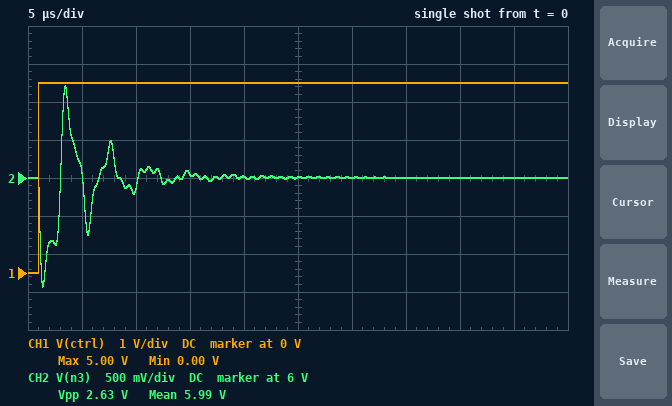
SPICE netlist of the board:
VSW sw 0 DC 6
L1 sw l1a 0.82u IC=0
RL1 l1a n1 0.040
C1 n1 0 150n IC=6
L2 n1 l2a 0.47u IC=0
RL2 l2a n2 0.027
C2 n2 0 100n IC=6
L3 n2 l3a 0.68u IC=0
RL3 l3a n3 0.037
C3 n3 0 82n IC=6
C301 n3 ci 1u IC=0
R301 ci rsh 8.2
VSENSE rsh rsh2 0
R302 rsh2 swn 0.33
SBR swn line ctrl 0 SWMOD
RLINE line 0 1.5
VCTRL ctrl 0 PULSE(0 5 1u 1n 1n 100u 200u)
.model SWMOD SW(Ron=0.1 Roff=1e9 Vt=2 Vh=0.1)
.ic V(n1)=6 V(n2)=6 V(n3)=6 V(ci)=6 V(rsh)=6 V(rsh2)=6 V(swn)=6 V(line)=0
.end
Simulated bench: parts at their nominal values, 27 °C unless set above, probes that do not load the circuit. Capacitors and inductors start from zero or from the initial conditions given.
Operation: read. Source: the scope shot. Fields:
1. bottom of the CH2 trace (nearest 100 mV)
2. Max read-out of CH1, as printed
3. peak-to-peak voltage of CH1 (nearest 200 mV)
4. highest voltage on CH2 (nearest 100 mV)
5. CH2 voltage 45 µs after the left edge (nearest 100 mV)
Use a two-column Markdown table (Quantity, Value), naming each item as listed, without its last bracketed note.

| Quantity | Value |
|---|---|
| bottom of the CH2 trace | 4.6 V |
| Max read-out of CH1, as printed | 5.00 V |
| peak-to-peak voltage of CH1 | 5.0 V |
| highest voltage on CH2 | 7.2 V |
| CH2 voltage 45 µs after the left edge | 6.0 V |
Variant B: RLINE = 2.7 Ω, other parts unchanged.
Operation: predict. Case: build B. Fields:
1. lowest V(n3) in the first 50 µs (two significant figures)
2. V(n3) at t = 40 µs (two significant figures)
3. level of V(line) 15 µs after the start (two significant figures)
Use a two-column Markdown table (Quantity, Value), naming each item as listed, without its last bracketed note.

| Quantity | Value |
|---|---|
| lowest V(n3) in the first 50 µs | 4.7 V |
| V(n3) at t = 40 µs | 6.0 V |
| level of V(line) 15 µs after the start | 430 mV |
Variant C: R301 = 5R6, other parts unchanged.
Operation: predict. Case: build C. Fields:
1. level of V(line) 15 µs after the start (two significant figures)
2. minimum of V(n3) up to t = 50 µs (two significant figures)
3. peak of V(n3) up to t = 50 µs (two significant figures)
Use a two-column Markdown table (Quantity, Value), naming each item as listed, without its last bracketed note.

| Quantity | Value |
|---|---|
| level of V(line) 15 µs after the start | 190 mV |
| minimum of V(n3) up to t = 50 µs | 4.2 V |
| peak of V(n3) up to t = 50 µs | 7.4 V |
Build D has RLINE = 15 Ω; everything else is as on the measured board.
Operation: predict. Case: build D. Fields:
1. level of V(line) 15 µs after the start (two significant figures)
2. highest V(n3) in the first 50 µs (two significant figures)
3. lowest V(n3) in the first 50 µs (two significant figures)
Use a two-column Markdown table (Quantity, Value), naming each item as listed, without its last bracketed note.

| Quantity | Value |
|---|---|
| level of V(line) 15 µs after the start | 2.2 V |
| highest V(n3) in the first 50 µs | 6.7 V |
| lowest V(n3) in the first 50 µs | 5.3 V |
